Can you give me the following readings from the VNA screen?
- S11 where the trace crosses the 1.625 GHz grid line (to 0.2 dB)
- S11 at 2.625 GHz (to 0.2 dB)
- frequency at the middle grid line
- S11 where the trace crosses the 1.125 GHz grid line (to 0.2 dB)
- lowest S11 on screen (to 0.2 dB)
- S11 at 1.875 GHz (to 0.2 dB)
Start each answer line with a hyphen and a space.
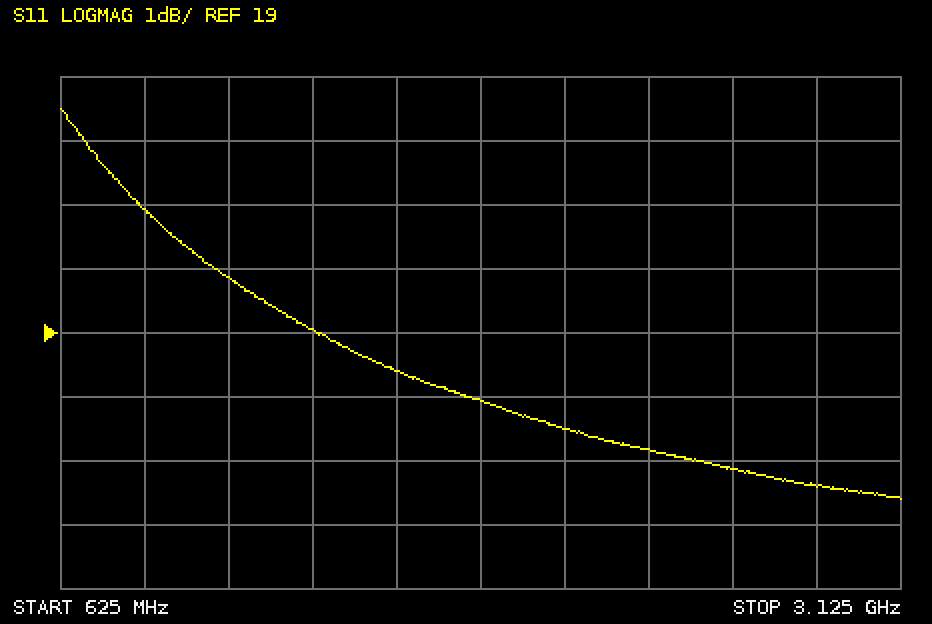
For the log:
- 18.4 dB
- 16.8 dB
- 1.875 GHz
- 19.8 dB
- 16.4 dB
- 18.0 dB
